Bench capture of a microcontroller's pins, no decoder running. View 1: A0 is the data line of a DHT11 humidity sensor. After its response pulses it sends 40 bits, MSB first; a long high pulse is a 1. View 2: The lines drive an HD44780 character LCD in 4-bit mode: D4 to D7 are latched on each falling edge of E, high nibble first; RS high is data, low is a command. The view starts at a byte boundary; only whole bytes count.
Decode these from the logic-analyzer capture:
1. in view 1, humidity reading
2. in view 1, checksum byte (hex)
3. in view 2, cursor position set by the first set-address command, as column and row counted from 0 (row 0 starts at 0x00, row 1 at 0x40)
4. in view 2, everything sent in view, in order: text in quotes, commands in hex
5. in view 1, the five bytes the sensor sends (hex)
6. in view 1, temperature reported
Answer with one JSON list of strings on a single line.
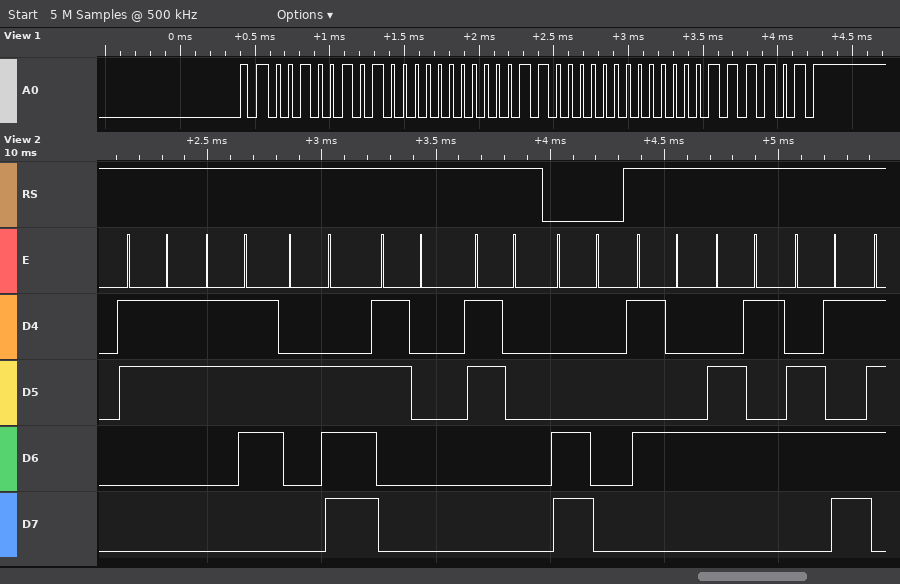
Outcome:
["37 %", "0x3D", "column 0, row 1", "\"37.00\" 0xC0 \"Tem\"", "25 00 18 00 3D", "24.0 °C"]
